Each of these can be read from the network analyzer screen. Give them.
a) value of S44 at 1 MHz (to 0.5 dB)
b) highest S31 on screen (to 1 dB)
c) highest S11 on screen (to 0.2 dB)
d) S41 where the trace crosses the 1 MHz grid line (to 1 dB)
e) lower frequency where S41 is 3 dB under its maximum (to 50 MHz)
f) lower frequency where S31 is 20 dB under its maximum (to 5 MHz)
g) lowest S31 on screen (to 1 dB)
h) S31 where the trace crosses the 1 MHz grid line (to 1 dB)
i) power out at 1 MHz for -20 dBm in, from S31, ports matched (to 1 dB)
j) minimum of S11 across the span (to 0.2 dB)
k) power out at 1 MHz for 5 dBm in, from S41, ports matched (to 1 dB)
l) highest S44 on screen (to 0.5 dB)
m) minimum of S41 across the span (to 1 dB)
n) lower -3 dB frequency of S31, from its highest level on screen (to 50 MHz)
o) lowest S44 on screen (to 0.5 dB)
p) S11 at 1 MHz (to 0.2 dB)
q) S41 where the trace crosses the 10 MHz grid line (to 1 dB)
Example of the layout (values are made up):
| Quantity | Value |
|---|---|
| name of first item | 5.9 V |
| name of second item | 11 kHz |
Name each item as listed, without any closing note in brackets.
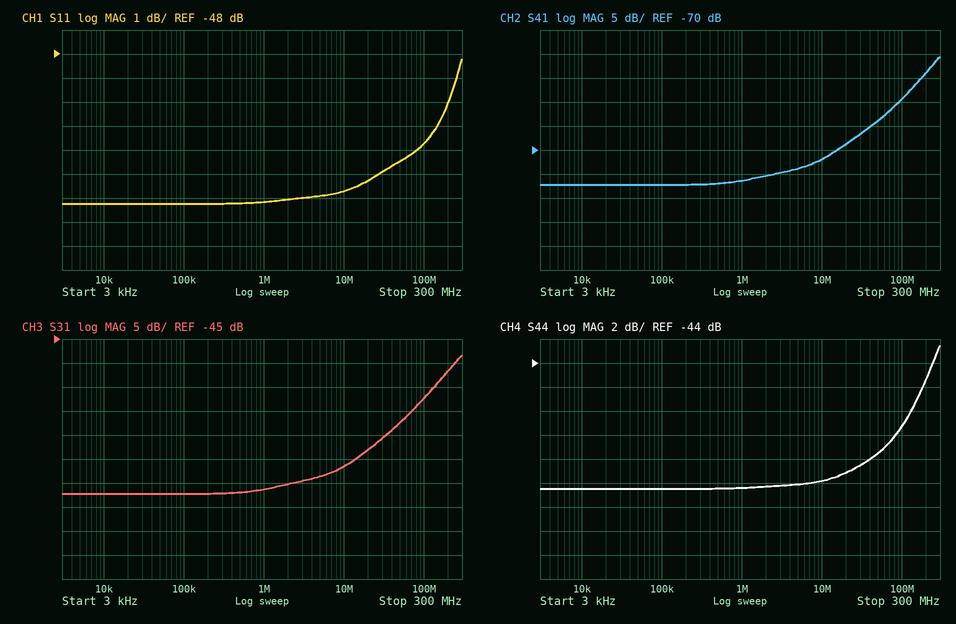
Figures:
| Quantity | Value |
|---|---|
| value of S44 at 1 MHz | -54.5 dB |
| highest S31 on screen | -48 dB |
| highest S11 on screen | -48.2 dB |
| S41 where the trace crosses the 1 MHz grid line | -76 dB |
| lower frequency where S41 is 3 dB under its maximum | 200 MHz |
| lower frequency where S31 is 20 dB under its maximum | 20 MHz |
| lowest S31 on screen | -77 dB |
| S31 where the trace crosses the 1 MHz grid line | -76 dB |
| power out at 1 MHz for -20 dBm in, from S31, ports matched | -96 dBm |
| minimum of S11 across the span | -54.2 dB |
| power out at 1 MHz for 5 dBm in, from S41, ports matched | -71 dBm |
| highest S44 on screen | -42.5 dB |
| minimum of S41 across the span | -77 dB |
| lower -3 dB frequency of S31, from its highest level on screen | 200 MHz |
| lowest S44 on screen | -54.5 dB |
| S11 at 1 MHz | -54.2 dB |
| S41 where the trace crosses the 10 MHz grid line | -72 dB |
